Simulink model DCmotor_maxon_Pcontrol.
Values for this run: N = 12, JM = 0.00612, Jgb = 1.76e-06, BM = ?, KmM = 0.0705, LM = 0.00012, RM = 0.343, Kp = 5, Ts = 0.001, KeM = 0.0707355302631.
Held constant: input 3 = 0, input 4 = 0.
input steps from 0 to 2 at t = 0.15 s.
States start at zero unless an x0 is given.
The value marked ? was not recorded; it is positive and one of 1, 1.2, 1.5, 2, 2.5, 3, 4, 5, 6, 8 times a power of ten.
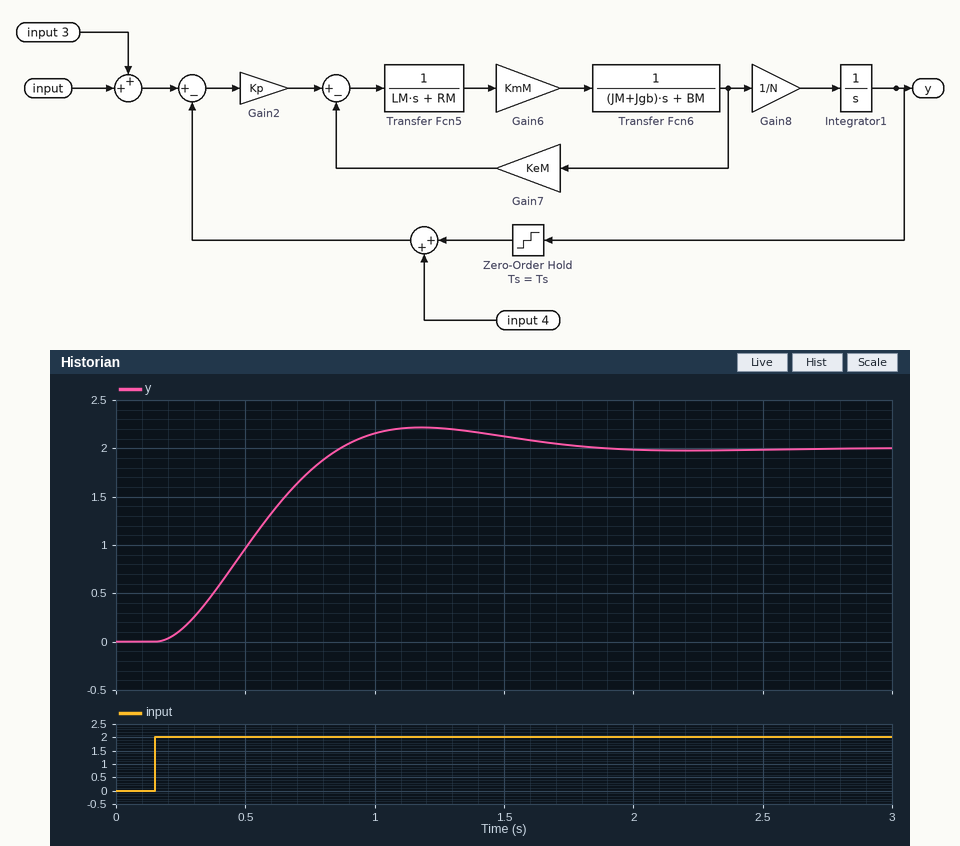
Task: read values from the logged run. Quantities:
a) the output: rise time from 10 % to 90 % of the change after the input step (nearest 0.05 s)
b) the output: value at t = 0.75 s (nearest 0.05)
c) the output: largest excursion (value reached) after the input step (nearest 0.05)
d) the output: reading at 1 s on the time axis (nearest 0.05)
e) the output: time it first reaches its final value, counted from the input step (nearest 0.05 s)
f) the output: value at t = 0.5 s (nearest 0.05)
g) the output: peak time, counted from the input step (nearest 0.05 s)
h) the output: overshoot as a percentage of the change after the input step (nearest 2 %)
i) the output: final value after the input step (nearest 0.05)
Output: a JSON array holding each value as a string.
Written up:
["0.50 s", "1.75", "2.20", "2.15", "0.70 s", "0.95", "1.05 s", "10 %", "2.00"]
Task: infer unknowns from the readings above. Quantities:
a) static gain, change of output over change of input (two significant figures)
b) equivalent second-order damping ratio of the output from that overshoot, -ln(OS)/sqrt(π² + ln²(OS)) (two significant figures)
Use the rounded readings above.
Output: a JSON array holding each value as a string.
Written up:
["1.0", "0.59"]
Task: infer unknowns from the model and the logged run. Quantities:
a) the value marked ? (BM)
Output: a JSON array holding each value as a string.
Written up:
["0.012"]
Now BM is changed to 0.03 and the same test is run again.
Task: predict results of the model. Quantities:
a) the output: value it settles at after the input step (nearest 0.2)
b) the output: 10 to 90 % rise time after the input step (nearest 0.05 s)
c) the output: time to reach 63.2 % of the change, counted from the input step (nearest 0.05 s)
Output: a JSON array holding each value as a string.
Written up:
["2.0", "0.85 s", "0.55 s"]
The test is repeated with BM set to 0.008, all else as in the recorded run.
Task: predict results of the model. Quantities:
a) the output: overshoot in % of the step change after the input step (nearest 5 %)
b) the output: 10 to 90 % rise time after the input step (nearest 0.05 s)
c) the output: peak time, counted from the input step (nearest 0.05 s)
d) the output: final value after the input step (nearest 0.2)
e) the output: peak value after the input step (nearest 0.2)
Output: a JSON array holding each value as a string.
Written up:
["15 %", "0.45 s", "0.95 s", "2.0", "2.4"]
